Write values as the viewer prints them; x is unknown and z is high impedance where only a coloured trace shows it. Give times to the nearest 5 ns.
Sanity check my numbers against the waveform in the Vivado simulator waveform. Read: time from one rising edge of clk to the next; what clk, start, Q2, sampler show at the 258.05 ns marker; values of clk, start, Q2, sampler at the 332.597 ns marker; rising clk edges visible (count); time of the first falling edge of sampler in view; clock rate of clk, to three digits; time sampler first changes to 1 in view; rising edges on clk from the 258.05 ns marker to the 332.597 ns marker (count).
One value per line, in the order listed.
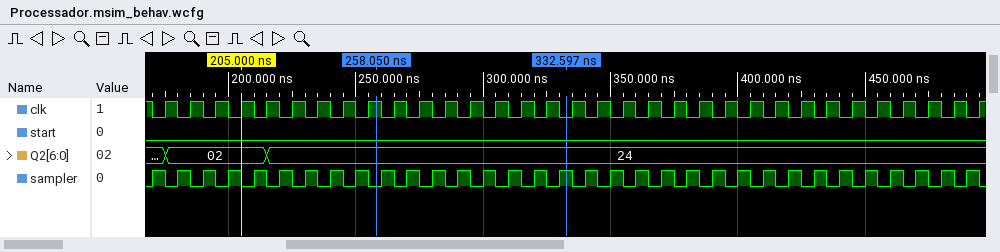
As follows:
10 ns
clk=1, start=0, Q2=24, sampler=0
clk=0, start=0, Q2=24, sampler=1
33
175 ns
100 MHz
170 ns
7
